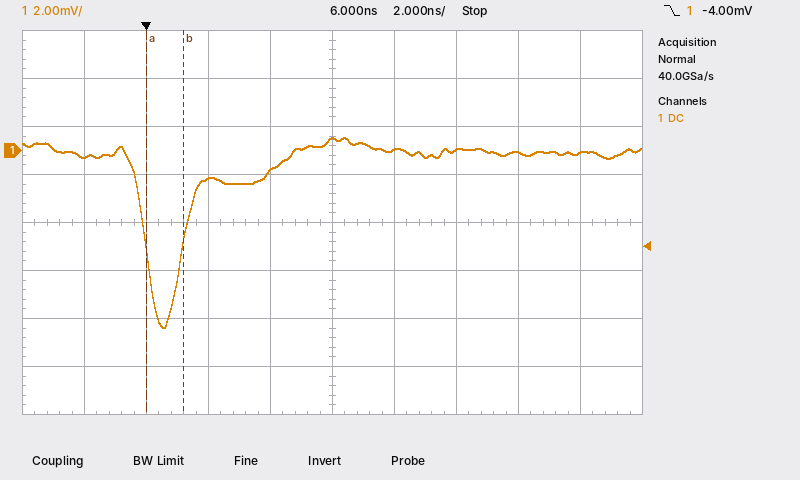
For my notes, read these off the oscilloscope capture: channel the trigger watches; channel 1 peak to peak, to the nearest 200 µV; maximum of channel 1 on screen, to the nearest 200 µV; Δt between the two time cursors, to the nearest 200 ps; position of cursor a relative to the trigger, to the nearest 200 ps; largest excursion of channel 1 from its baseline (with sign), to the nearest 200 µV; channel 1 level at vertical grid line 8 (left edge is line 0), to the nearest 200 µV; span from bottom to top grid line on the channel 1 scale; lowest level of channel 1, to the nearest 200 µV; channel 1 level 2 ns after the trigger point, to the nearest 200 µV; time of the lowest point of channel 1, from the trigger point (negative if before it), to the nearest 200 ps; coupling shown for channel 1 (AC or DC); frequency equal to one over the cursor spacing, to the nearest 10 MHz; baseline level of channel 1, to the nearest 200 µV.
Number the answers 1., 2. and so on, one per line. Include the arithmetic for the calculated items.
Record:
1. channel 1
2. 600 µV − (-7.4 mV) = 8.0 mV
3. 600 µV
4. 1.2 ns
5. 0.0 ns
6. -7.4 mV − (0.0 mV) = -7.4 mV
7. 0.0 mV
8. 16 mV
9. -7.4 mV
10. -1.2 mV
11. +600 ps
12. DC
13. 1 / 1.2 ns ≈ 830 MHz
14. 0.0 mV
